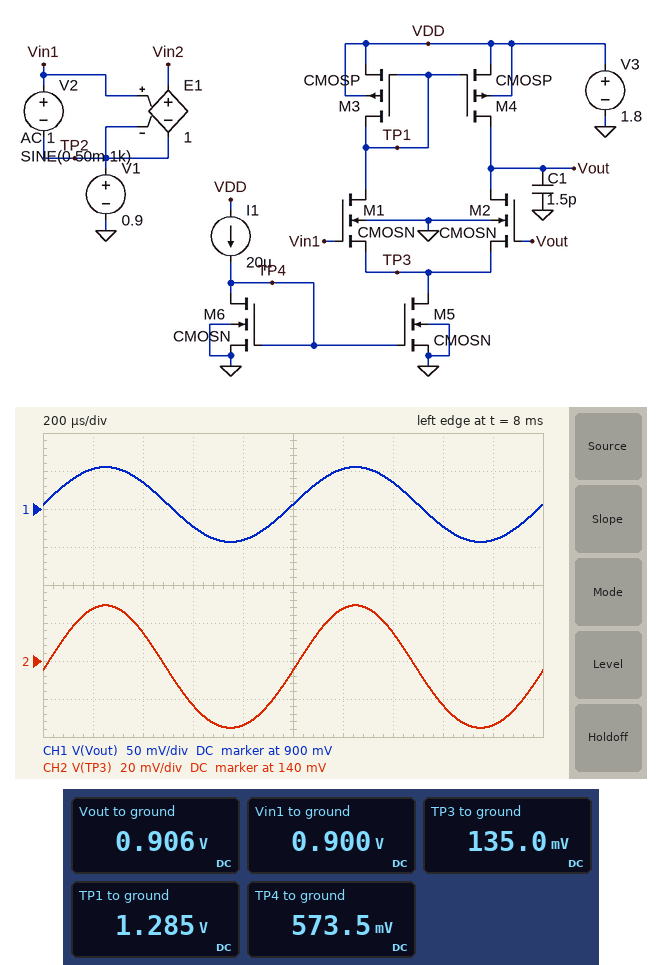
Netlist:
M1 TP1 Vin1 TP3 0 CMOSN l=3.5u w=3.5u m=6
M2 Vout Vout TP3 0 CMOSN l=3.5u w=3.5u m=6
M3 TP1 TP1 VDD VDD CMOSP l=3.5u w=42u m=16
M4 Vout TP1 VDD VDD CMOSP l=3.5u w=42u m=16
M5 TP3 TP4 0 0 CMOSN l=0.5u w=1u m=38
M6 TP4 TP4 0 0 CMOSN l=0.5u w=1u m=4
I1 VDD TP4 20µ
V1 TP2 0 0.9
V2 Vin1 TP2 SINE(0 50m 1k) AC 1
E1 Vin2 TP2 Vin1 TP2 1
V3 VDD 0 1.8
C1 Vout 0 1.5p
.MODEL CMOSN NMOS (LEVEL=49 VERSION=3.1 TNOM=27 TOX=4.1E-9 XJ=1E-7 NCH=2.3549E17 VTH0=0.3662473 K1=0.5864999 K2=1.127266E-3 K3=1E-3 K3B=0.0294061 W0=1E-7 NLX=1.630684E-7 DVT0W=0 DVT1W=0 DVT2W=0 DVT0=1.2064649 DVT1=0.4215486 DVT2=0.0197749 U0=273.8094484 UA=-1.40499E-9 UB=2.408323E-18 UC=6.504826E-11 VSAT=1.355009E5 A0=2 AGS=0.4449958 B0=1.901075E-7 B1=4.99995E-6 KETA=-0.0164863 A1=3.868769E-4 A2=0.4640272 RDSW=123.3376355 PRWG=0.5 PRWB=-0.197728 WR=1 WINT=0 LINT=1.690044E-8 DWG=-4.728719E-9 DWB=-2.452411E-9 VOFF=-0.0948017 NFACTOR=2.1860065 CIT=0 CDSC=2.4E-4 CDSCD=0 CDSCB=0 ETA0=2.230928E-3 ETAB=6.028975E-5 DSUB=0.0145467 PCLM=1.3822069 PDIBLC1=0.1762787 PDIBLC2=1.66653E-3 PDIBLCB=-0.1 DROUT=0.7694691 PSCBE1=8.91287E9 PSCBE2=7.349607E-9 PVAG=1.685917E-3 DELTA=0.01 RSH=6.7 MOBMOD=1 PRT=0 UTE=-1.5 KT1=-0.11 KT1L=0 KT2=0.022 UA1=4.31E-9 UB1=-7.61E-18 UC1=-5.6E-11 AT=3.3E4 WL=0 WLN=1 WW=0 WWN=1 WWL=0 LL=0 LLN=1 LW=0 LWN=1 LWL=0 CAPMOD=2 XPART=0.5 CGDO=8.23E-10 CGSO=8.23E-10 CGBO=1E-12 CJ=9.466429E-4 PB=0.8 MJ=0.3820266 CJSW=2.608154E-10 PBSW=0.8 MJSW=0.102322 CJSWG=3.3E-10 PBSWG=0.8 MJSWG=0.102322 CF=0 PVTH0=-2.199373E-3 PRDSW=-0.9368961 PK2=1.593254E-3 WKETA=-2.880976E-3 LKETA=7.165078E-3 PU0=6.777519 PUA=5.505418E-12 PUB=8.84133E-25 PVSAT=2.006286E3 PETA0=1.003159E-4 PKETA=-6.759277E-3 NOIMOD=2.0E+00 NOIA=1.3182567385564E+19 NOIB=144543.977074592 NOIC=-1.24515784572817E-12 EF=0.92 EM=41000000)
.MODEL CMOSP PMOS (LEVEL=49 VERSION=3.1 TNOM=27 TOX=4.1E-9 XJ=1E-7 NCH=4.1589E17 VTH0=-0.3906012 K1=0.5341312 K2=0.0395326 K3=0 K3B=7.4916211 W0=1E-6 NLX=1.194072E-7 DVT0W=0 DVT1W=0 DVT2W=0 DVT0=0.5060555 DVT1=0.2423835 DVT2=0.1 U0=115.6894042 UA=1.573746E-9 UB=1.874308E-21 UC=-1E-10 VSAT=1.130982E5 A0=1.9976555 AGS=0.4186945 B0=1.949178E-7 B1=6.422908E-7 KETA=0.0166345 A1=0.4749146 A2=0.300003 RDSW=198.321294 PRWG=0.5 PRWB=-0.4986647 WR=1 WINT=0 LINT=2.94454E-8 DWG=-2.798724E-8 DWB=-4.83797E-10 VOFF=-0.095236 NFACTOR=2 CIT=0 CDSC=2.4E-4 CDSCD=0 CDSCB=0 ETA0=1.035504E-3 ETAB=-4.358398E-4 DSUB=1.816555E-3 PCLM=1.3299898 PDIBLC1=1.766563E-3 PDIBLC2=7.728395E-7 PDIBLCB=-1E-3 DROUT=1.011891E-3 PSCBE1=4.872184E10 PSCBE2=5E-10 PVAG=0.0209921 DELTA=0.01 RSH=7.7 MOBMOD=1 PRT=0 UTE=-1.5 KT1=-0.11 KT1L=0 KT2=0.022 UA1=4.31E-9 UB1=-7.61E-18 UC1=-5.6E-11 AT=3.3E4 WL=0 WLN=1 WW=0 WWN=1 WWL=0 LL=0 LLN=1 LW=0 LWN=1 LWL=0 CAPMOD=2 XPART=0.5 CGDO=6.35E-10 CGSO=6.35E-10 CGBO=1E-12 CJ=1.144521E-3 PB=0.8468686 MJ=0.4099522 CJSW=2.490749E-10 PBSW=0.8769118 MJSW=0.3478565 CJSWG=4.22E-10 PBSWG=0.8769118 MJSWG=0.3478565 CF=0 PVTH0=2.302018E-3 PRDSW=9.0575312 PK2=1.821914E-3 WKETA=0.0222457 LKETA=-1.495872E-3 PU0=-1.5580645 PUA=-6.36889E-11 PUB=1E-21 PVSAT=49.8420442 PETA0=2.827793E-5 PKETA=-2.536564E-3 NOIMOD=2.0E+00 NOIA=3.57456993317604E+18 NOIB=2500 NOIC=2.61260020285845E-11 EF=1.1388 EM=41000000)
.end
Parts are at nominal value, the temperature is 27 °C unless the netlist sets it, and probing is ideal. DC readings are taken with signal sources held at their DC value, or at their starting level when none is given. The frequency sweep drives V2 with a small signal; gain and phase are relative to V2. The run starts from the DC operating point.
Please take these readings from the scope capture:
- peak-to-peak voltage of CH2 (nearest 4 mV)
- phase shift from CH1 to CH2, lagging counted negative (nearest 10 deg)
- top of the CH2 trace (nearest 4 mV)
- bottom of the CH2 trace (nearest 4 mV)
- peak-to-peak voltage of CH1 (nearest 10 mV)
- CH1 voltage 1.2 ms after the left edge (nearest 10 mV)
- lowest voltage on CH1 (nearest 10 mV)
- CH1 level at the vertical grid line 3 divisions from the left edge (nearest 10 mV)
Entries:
64 mV
0 deg
168 mV
104 mV
100 mV
950 mV
860 mV
880 mV
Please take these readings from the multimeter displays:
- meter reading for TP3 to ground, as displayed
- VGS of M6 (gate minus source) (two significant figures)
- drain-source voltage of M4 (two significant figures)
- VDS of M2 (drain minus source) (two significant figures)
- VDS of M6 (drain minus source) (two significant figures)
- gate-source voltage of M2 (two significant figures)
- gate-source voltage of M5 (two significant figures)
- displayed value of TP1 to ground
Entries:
135.0 mV
570 mV
-890 mV
770 mV
570 mV
770 mV
570 mV
1.285 V
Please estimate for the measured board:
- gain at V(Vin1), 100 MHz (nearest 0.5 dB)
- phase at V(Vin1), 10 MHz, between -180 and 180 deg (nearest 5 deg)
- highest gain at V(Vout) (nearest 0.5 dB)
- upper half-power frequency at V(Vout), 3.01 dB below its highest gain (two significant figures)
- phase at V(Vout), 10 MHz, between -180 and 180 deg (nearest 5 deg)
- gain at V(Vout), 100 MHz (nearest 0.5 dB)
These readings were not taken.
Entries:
0 dB
0 deg
0 dB
15 MHz
-40 deg
-22.5 dB
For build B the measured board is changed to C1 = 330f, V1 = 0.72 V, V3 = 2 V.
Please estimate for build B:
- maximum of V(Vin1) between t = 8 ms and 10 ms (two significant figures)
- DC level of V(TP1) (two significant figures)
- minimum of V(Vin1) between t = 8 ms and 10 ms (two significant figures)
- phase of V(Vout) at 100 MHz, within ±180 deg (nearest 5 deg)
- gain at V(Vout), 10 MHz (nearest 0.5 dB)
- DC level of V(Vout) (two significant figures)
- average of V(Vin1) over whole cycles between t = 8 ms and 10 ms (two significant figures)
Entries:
770 mV
1.5 V
670 mV
35 deg
-5.5 dB
730 mV
720 mV
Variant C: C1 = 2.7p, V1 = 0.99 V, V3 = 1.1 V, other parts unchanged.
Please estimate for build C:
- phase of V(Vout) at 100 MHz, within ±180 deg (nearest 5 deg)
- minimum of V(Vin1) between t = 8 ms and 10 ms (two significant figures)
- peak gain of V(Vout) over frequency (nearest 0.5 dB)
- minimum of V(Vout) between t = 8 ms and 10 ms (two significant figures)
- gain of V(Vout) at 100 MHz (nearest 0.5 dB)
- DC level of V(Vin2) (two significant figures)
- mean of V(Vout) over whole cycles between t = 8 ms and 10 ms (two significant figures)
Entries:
-70 deg
940 mV
-2.0 dB
930 mV
-26.0 dB
990 mV
970 mV
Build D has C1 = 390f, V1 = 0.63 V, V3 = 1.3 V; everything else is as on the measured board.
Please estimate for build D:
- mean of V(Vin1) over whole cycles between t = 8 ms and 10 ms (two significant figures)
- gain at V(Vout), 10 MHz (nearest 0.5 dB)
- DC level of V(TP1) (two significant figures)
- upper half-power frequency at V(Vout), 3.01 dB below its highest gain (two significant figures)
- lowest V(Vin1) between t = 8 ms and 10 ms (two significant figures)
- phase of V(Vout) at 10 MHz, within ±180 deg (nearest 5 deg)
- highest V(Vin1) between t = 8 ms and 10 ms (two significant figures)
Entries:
630 mV
-8.5 dB
840 mV
4.4 MHz
580 mV
-95 deg
680 mV
